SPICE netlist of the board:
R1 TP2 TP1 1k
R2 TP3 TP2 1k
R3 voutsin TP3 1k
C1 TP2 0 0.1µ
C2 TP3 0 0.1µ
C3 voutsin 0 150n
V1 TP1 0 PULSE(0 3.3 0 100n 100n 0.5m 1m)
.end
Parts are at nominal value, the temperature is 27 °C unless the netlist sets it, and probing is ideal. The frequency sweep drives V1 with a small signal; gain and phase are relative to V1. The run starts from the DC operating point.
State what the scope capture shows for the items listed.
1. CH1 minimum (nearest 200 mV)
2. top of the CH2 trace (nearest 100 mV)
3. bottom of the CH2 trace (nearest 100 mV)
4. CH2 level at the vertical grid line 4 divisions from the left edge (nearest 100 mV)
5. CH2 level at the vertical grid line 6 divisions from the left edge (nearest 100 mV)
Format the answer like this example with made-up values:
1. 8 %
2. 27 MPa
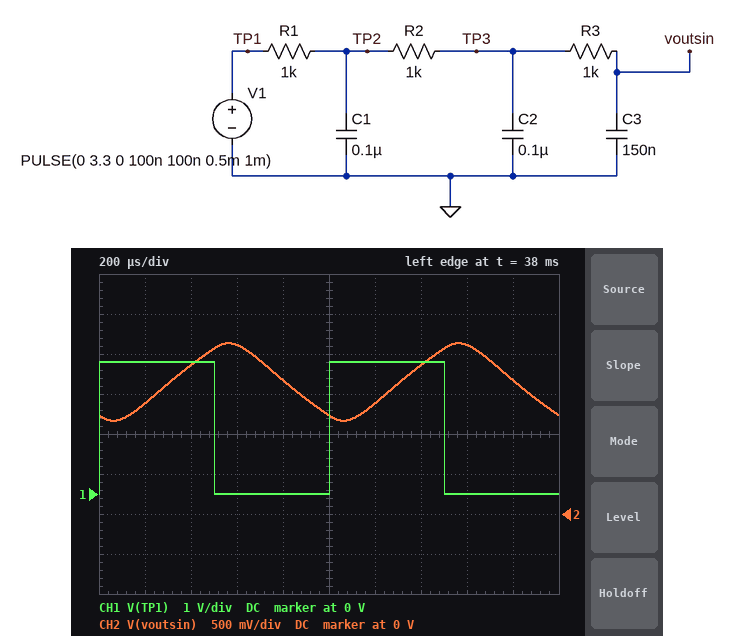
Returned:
1. 0 V
2. 2.1 V
3. 1.2 V
4. 1.7 V
5. 1.4 V
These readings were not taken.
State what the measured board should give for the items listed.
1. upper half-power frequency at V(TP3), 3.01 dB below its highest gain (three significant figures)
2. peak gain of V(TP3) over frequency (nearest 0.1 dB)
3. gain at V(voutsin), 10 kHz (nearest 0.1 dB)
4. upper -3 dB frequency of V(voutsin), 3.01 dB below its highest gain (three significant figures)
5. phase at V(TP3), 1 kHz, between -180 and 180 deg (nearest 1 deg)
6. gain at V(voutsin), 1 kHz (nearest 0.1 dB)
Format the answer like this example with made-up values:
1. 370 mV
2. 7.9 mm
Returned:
1. 257 Hz
2. 0 dB
3. -52.6 dB
4. 243 Hz
5. -69 deg
6. -13.4 dB
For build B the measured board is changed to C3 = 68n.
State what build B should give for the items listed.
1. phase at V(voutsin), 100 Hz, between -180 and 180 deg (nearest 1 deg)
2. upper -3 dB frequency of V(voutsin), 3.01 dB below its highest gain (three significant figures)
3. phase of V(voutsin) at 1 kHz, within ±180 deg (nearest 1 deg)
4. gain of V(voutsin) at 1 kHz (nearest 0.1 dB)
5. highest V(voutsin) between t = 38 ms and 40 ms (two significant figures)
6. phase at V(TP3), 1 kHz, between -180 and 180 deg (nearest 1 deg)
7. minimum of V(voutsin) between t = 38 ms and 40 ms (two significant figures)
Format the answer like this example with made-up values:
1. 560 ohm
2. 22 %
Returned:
1. -18 deg
2. 372 Hz
3. -99 deg
4. -9.6 dB
5. 2.4 V
6. -76 deg
7. 900 mV
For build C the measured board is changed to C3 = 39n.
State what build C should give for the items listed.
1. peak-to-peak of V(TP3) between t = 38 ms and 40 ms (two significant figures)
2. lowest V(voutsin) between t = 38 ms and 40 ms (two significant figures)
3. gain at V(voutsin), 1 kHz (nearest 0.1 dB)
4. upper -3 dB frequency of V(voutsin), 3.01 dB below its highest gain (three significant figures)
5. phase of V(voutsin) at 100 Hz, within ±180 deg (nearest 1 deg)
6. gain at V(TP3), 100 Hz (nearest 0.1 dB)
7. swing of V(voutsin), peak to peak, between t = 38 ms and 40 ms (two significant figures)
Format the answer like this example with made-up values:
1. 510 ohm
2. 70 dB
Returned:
1. 1.9 V
2. 740 mV
3. -8.0 dB
4. 450 Hz
5. -15 deg
6. -0.2 dB
7. 1.8 V
